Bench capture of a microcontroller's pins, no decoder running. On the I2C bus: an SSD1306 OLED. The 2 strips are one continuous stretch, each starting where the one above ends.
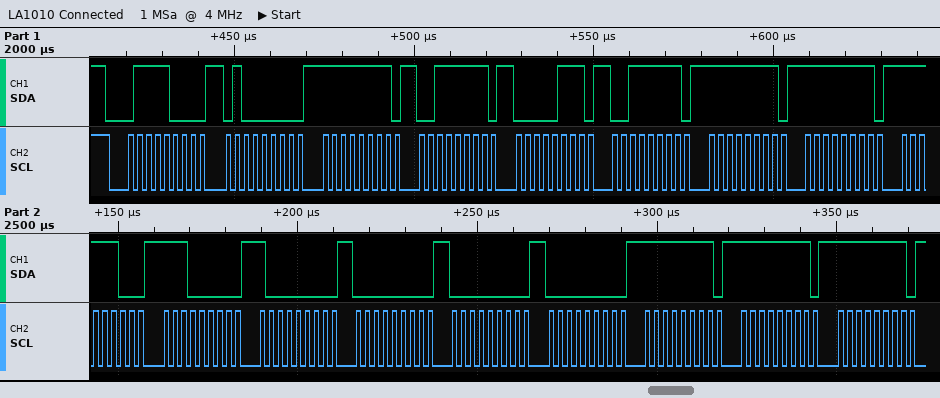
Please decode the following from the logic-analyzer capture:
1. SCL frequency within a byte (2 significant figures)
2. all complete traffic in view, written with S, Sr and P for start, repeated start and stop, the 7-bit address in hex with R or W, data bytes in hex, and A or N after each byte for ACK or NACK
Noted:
400 kHz
S 3CW A 40 A FF A 3F A 07 A 3F A FF A FF A FC A E0 A 80 A 00 A 00 A 00 A FF A FF A FF A
